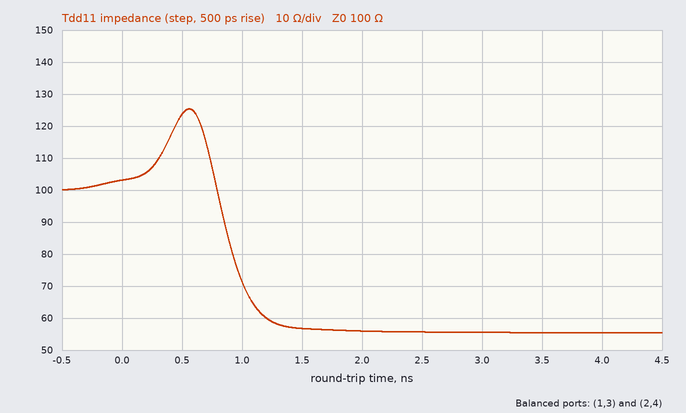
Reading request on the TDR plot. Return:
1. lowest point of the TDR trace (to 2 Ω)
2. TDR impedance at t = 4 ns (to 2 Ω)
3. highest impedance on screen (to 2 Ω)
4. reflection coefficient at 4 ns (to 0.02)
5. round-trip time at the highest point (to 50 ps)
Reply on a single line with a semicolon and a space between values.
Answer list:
56 Ω; 56 Ω; 126 Ω; -0.28; 550 ps
